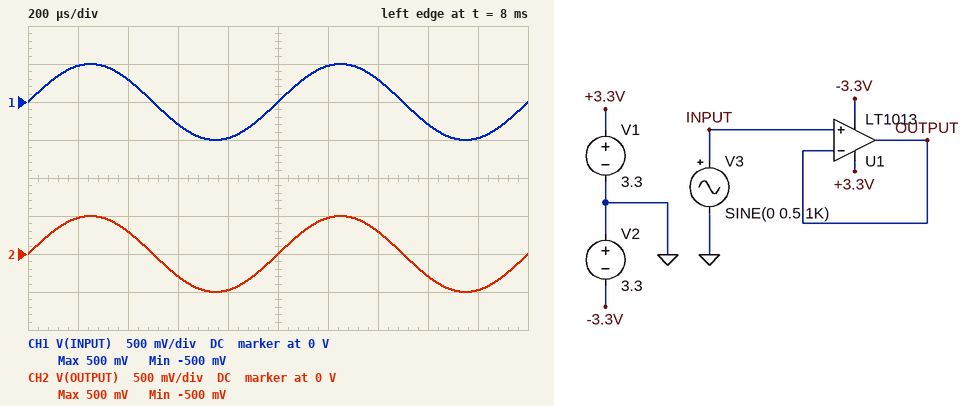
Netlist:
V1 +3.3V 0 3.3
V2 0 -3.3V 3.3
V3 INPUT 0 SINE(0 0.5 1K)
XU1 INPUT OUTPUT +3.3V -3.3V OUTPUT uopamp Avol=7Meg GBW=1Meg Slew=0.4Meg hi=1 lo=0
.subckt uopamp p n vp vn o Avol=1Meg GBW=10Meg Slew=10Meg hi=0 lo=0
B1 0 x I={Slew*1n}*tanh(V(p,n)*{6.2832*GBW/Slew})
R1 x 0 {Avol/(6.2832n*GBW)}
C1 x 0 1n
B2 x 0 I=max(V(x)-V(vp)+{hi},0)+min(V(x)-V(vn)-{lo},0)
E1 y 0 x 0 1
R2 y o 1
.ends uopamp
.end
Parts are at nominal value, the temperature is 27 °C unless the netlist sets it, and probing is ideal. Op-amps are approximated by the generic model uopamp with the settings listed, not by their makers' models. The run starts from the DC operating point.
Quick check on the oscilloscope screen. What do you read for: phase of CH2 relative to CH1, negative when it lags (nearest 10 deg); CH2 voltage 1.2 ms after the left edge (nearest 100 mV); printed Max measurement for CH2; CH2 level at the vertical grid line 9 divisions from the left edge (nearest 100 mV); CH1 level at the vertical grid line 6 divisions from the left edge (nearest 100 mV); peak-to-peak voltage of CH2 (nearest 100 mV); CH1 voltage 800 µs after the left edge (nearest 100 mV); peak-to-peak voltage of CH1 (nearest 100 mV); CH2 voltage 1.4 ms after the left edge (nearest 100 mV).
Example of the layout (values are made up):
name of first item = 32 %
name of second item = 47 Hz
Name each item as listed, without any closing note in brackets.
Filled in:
phase of CH2 relative to CH1, negative when it lags = 0 deg
CH2 voltage 1.2 ms after the left edge = 500 mV
printed Max measurement for CH2 = 500 mV
CH2 level at the vertical grid line 9 divisions from the left edge = -500 mV
CH1 level at the vertical grid line 6 divisions from the left edge = 500 mV
peak-to-peak voltage of CH2 = 1.0 V
CH1 voltage 800 µs after the left edge = -500 mV
peak-to-peak voltage of CH1 = 1.0 V
CH2 voltage 1.4 ms after the left edge = 300 mV
